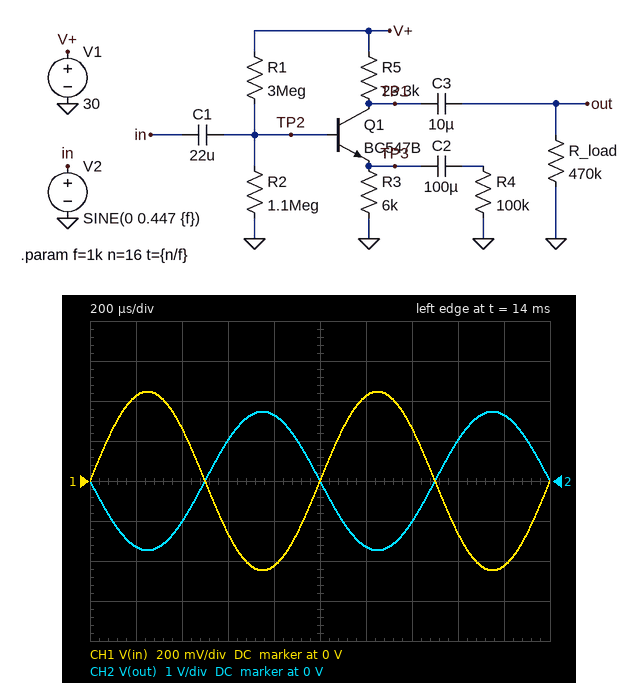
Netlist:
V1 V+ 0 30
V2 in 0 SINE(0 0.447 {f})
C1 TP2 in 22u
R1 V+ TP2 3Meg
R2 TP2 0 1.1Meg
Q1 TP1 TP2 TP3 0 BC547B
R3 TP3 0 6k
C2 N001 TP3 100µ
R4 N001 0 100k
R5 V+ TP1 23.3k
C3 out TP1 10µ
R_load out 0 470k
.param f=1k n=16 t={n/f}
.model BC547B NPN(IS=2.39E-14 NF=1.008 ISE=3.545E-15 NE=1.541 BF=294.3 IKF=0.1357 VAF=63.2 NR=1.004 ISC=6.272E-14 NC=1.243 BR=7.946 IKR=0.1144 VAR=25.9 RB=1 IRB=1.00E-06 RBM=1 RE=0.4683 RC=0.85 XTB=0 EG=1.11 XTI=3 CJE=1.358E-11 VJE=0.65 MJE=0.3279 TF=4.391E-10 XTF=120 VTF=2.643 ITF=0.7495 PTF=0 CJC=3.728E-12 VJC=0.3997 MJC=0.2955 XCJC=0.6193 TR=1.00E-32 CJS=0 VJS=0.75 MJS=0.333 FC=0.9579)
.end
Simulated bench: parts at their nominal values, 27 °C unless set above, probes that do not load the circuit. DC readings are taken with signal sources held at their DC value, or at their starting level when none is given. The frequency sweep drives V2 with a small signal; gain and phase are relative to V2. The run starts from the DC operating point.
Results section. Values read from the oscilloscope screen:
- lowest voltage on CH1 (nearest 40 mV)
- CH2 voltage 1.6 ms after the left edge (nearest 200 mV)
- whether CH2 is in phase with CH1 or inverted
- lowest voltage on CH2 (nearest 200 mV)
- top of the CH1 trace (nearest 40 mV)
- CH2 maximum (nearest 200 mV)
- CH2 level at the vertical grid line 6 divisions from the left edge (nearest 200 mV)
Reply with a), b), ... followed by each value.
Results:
a) -440 mV
b) 1.0 V
c) inverted
d) -1.8 V
e) 440 mV
f) 1.8 V
g) -1.6 V
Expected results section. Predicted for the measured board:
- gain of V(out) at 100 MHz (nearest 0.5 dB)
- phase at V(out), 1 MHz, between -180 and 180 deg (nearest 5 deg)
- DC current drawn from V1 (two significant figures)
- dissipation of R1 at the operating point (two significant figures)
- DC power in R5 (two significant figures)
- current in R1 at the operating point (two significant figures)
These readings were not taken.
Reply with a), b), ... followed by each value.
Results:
a) 0.5 dB
b) 160 deg
c) 860 µA
d) 200 µW
e) 17 mW
f) 8.1 µA
